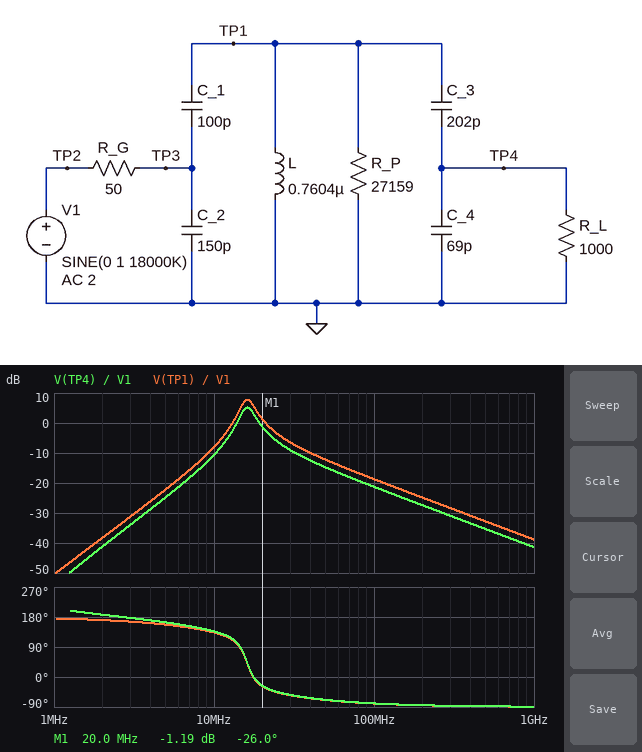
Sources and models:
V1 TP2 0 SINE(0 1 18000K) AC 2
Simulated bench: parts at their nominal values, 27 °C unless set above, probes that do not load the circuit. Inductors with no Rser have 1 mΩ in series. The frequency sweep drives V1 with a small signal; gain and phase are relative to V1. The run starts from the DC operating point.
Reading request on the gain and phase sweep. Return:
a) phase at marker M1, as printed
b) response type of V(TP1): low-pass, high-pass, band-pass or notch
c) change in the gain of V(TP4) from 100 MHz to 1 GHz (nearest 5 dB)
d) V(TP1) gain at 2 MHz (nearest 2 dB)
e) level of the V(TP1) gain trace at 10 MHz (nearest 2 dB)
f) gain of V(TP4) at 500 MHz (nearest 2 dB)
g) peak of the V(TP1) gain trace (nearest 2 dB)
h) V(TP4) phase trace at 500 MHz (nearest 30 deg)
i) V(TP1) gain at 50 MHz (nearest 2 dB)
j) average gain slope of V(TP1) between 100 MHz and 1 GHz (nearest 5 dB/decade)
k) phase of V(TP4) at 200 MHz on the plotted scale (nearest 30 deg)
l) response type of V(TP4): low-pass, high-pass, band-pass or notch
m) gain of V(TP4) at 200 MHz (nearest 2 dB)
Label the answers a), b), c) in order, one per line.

a) -26.0 deg
b) band-pass
c) -20 dB
d) -38 dB
e) -8 dB
f) -36 dB
g) 8 dB
h) -90 deg
i) -12 dB
j) -20 dB/decade
k) -90 deg
l) band-pass
m) -28 dB
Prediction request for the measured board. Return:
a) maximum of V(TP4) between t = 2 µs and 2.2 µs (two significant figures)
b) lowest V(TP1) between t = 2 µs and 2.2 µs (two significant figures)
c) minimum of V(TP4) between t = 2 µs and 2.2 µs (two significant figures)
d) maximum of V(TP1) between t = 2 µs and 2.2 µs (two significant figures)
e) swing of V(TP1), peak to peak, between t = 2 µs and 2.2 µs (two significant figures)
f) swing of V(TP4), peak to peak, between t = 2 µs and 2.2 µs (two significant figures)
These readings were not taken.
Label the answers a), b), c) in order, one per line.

a) 1.3 V
b) -1.8 V
c) -1.3 V
d) 1.8 V
e) 3.5 V
f) 2.6 V
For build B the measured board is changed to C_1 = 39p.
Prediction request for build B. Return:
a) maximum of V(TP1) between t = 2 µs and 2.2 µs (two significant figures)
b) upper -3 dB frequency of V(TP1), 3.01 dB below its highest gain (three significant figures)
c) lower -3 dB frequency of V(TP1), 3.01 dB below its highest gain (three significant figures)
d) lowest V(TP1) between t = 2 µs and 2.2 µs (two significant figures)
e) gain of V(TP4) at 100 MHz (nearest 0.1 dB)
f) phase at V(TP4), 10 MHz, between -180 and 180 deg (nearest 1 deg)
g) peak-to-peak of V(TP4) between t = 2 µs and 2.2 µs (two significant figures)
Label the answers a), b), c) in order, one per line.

a) 1.4 V
b) 20.8 MHz
c) 18.7 MHz
d) -1.4 V
e) -24.3 dB
f) 150 deg
g) 2.1 V
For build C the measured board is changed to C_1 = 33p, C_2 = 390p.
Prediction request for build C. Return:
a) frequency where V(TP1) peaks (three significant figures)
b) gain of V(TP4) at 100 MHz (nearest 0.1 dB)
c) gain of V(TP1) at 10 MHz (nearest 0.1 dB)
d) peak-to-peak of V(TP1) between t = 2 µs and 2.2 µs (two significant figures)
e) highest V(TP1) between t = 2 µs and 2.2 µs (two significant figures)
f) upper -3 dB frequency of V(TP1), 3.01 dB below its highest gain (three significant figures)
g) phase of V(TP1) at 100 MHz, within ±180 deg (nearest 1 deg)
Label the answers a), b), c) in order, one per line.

a) 20.1 MHz
b) -32.6 dB
c) -22.0 dB
d) 1.2 V
e) 600 mV
f) 20.8 MHz
g) -85 deg
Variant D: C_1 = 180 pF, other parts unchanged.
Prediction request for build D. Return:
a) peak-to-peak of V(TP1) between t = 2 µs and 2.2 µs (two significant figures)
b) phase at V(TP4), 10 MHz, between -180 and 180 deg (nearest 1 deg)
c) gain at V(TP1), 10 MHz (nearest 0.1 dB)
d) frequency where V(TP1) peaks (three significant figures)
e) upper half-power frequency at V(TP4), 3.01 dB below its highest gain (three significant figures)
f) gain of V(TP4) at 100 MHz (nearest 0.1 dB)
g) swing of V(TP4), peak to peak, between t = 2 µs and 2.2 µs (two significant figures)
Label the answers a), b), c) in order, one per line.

a) 2.4 V
b) 116 deg
c) -2.3 dB
d) 14.1 MHz
e) 17.1 MHz
f) -20.2 dB
g) 1.8 V
